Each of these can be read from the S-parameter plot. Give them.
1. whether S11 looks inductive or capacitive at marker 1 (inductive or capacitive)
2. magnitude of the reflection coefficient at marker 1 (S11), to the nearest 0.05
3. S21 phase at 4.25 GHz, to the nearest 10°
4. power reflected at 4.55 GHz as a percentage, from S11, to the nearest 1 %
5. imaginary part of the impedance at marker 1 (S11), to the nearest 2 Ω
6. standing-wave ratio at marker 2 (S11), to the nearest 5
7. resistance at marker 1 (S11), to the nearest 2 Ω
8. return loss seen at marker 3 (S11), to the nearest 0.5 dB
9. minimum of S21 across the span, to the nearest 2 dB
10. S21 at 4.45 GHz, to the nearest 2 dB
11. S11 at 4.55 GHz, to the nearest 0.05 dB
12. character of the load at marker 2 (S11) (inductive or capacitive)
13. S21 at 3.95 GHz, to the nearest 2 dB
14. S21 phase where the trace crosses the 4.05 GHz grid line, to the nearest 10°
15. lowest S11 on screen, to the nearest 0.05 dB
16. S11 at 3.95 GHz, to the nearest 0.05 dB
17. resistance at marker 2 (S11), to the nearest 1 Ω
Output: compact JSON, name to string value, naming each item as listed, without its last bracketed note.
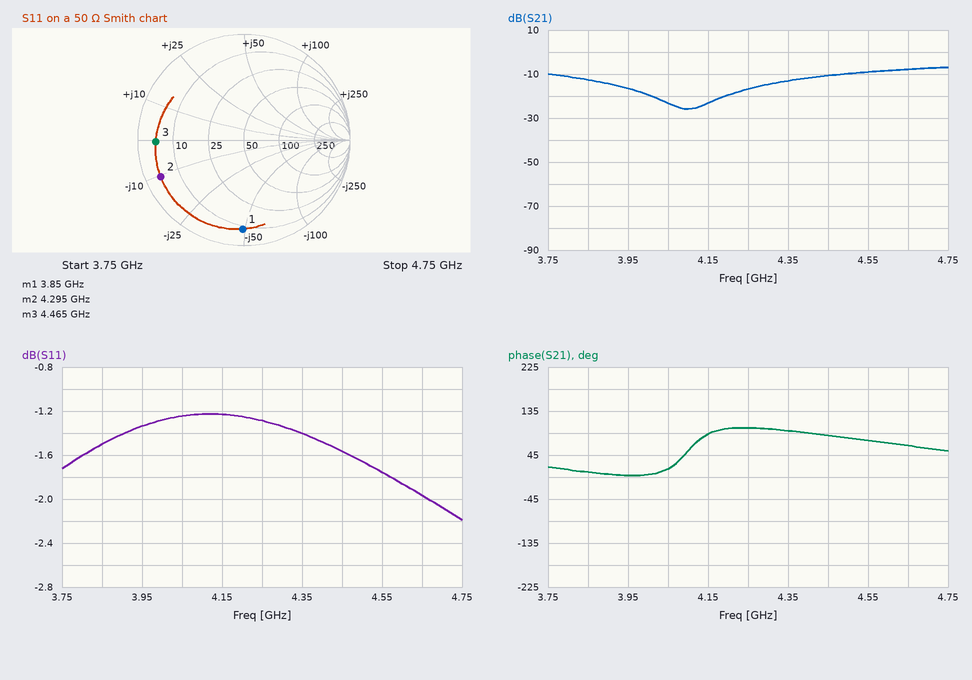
{"whether S11 looks inductive or capacitive at marker 1": "capacitive", "magnitude of the reflection coefficient at marker 1 (S11), to the nearest 0.05": "0.85", "S21 phase at 4.25 GHz, to the nearest 10°": "100°", "power reflected at 4.55 GHz as a percentage, from S11, to the nearest 1 %": "67 %", "imaginary part of the impedance at marker 1 (S11), to the nearest 2 Ω": "-48 Ω", "standing-wave ratio at marker 2 (S11), to the nearest 5": "15", "resistance at marker 1 (S11), to the nearest 2 Ω": "8 Ω", "return loss seen at marker 3 (S11), to the nearest 0.5 dB": "1.5 dB", "minimum of S21 across the span, to the nearest 2 dB": "-26 dB", "S21 at 4.45 GHz, to the nearest 2 dB": "-10 dB", "S11 at 4.55 GHz, to the nearest 0.05 dB": "-1.75 dB", "character of the load at marker 2 (S11)": "capacitive", "S21 at 3.95 GHz, to the nearest 2 dB": "-16 dB", "S21 phase where the trace crosses the 4.05 GHz grid line, to the nearest 10°": "20°", "lowest S11 on screen, to the nearest 0.05 dB": "-2.20 dB", "S11 at 3.95 GHz, to the nearest 0.05 dB": "-1.35 dB", "resistance at marker 2 (S11), to the nearest 1 Ω": "4 Ω"}
